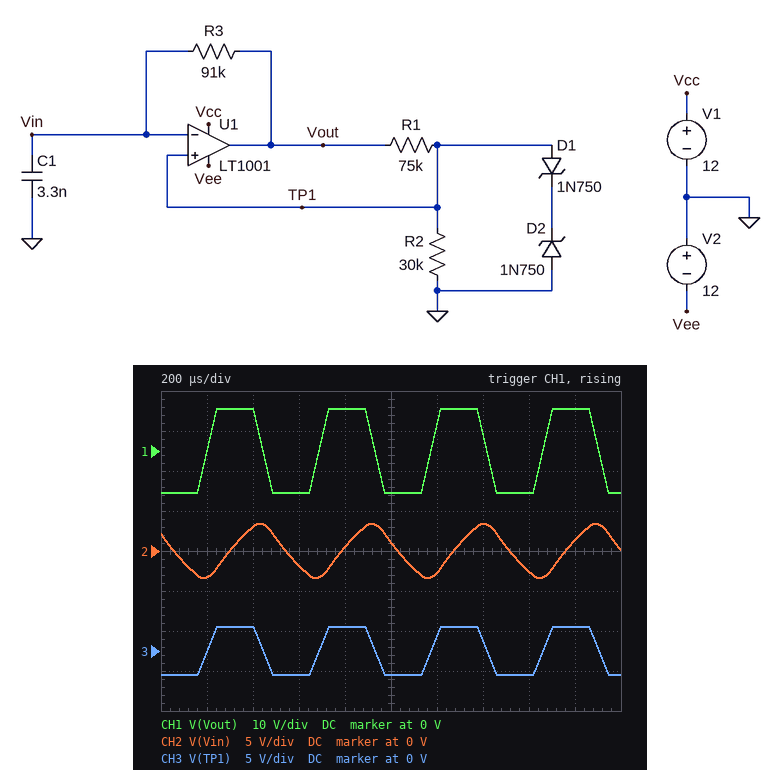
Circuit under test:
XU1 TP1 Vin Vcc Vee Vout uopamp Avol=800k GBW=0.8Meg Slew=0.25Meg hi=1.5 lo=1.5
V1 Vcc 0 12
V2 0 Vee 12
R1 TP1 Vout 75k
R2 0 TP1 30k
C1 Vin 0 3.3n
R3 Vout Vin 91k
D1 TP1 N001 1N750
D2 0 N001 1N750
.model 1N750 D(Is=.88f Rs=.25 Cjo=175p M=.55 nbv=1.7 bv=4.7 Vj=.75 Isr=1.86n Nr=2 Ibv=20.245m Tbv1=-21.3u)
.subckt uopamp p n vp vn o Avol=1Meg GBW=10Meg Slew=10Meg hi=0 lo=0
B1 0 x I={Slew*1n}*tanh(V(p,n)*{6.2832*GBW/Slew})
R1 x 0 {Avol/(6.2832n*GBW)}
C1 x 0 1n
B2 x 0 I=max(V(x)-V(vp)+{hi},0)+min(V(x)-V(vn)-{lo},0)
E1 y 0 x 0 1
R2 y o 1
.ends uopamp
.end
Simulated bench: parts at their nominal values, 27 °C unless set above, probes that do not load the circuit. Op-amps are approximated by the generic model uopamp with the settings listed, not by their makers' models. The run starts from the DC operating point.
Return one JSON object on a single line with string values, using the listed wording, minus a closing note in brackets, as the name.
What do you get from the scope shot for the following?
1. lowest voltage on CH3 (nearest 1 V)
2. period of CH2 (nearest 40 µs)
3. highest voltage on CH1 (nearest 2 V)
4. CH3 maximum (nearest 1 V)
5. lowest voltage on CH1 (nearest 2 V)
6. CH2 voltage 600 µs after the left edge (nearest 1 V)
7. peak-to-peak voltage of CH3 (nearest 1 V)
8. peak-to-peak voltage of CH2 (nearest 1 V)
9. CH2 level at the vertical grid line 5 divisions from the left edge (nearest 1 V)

{"lowest voltage on CH3": "-3 V", "period of CH2": "480 µs", "highest voltage on CH1": "10 V", "CH3 maximum": "3 V", "lowest voltage on CH1": "-10 V", "CH2 voltage 600 µs after the left edge": "-2 V", "peak-to-peak voltage of CH3": "6 V", "peak-to-peak voltage of CH2": "7 V", "CH2 level at the vertical grid line 5 divisions from the left edge": "1 V"}
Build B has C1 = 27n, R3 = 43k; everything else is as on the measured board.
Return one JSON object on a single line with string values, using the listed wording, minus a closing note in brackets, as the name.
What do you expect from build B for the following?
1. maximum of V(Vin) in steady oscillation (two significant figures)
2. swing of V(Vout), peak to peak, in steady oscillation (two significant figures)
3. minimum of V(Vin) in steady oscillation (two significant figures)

{"maximum of V(Vin) in steady oscillation": "3.1 V", "swing of V(Vout), peak to peak, in steady oscillation": "21 V", "minimum of V(Vin) in steady oscillation": "-3.1 V"}
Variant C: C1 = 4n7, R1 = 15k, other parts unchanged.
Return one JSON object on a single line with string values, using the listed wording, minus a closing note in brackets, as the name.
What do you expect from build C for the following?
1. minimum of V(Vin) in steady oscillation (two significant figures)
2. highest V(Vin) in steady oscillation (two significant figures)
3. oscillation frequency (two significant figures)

{"minimum of V(Vin) in steady oscillation": "-5.3 V", "highest V(Vin) in steady oscillation": "5.3 V", "oscillation frequency": "970 Hz"}
